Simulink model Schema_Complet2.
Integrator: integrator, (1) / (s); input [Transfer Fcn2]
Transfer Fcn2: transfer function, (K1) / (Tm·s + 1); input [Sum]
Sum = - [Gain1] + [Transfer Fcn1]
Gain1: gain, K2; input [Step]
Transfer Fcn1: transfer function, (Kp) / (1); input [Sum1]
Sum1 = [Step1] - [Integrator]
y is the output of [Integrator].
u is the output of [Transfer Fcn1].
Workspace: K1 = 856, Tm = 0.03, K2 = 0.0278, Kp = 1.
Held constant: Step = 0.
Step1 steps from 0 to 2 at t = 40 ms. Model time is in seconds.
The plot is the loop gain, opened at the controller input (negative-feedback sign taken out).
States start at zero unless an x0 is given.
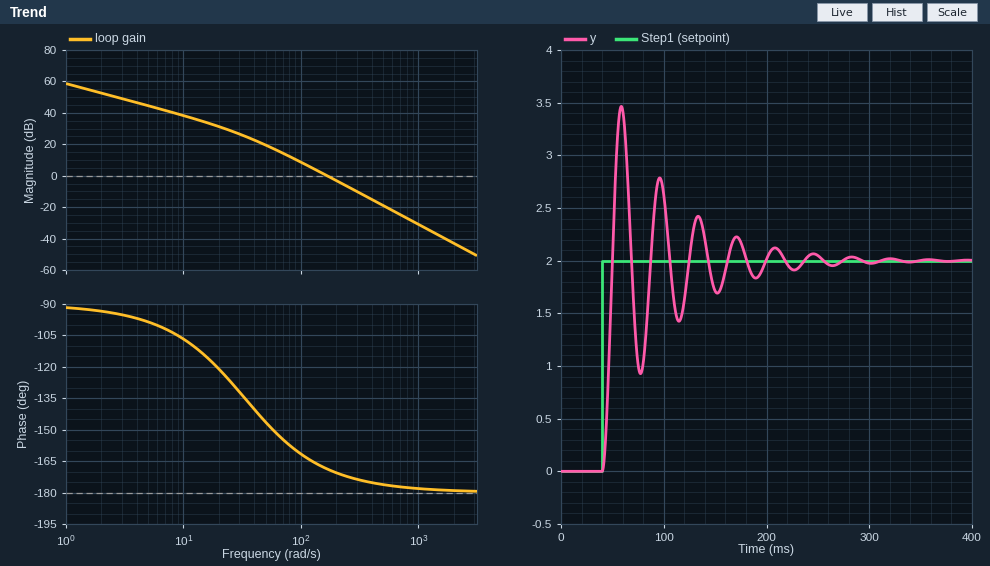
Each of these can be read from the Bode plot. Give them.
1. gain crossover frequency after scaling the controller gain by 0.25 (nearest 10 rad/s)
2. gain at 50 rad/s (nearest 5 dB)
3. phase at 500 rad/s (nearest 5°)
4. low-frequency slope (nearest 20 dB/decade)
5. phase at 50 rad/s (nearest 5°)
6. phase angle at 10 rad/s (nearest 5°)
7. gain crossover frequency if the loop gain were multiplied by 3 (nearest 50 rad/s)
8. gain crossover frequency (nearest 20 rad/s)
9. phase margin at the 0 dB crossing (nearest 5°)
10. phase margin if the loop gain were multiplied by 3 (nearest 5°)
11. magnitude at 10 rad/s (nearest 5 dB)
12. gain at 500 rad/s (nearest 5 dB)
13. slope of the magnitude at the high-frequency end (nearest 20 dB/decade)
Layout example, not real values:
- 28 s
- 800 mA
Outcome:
- 80 rad/s
- 20 dB
- -175°
- -20 dB/decade
- -145°
- -105°
- 300 rad/s
- 160 rad/s
- 10°
- 5°
- 40 dB
- -20 dB
- -40 dB/decade
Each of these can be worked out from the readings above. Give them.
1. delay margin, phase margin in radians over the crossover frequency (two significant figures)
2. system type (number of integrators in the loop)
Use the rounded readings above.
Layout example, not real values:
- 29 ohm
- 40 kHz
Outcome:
- 0.0011 s
- 1
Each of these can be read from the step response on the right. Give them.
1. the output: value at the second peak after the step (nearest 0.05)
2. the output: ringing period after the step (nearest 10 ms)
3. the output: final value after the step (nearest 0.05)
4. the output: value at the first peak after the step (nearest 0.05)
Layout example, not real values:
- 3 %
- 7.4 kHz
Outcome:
- 2.80
- 40 ms
- 2.00
- 3.45
